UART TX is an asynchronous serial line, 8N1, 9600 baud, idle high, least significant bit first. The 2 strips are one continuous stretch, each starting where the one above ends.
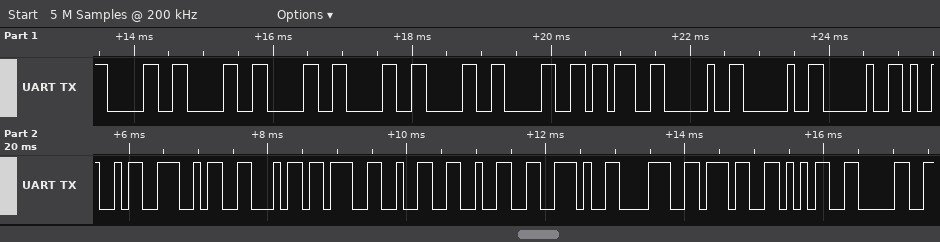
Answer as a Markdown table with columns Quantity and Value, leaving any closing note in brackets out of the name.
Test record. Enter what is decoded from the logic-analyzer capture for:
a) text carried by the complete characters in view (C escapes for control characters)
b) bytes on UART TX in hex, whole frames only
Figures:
| Quantity | Value |
|---|---|
| text carried by the complete characters in view | "000000;   INF;22.8750" |
| bytes on UART TX in hex, whole frames only | 30 30 30 30 30 30 3B 20 20 20 49 4E 46 3B 32 32 2E 38 37 35 30 |
